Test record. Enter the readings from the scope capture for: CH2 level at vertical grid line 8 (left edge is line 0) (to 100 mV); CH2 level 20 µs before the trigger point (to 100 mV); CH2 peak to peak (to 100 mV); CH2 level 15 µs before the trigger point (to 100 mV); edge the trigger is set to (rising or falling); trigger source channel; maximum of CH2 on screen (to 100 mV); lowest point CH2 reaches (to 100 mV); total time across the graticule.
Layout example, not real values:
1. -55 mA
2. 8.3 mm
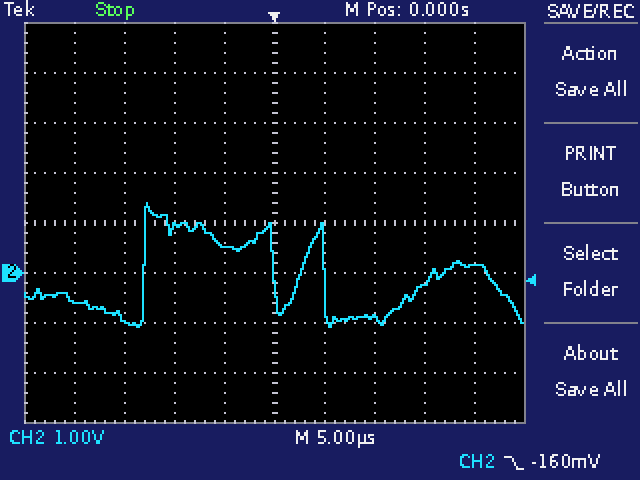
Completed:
1. -200 mV
2. -600 mV
3. 2.5 V
4. -900 mV
5. falling
6. CH2
7. 1.4 V
8. -1.1 V
9. 50 µs
